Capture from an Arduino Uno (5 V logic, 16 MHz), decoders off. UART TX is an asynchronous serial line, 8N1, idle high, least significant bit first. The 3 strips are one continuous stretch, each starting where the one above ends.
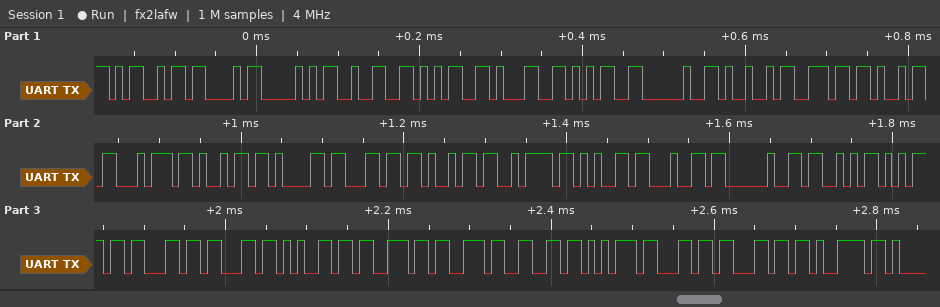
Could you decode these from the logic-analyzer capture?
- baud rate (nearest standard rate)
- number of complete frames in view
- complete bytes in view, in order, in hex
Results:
115200 baud
32
0x4D 0x43 0x50 0x32 0x35 0x31 0x35 0x20 0x49 0x6E 0x69 0x74 0x69 0x61 0x6C 0x69 0x7A 0x65 0x64 0x20 0x53 0x75 0x63 0x63 0x65 0x73 0x73 0x66 0x75 0x6C 0x6C 0x79
